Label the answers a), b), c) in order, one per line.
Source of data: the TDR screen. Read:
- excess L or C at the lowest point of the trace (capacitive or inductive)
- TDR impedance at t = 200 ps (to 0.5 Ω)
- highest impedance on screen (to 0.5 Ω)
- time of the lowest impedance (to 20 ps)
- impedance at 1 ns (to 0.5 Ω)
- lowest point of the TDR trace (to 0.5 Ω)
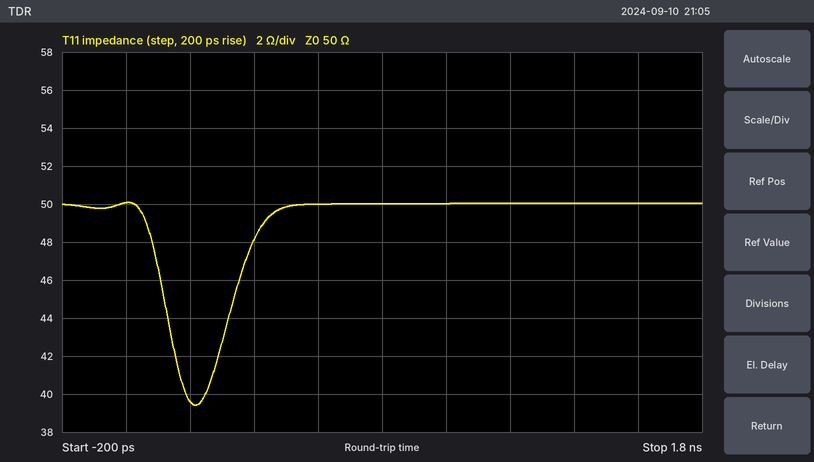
a) capacitive
b) 39.5 Ω
c) 50.0 Ω
d) 220 ps
e) 50.0 Ω
f) 39.5 Ω
